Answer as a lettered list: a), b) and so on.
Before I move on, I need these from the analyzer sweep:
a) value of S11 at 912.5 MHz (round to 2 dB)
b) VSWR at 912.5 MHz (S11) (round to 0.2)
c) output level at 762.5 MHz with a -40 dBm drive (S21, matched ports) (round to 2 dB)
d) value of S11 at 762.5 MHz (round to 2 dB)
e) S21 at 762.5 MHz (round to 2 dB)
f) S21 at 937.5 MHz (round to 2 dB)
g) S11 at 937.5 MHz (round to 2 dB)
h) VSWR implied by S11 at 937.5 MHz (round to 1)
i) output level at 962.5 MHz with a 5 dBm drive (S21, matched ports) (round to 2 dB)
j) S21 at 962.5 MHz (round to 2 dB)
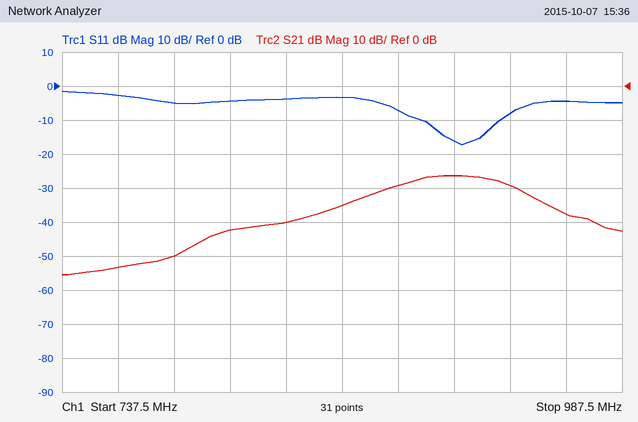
a) -16 dB
b) 1.4
c) -94 dBm
d) -2 dB
e) -54 dB
f) -30 dB
g) -8 dB
h) 2
i) -32 dBm
j) -38 dB
